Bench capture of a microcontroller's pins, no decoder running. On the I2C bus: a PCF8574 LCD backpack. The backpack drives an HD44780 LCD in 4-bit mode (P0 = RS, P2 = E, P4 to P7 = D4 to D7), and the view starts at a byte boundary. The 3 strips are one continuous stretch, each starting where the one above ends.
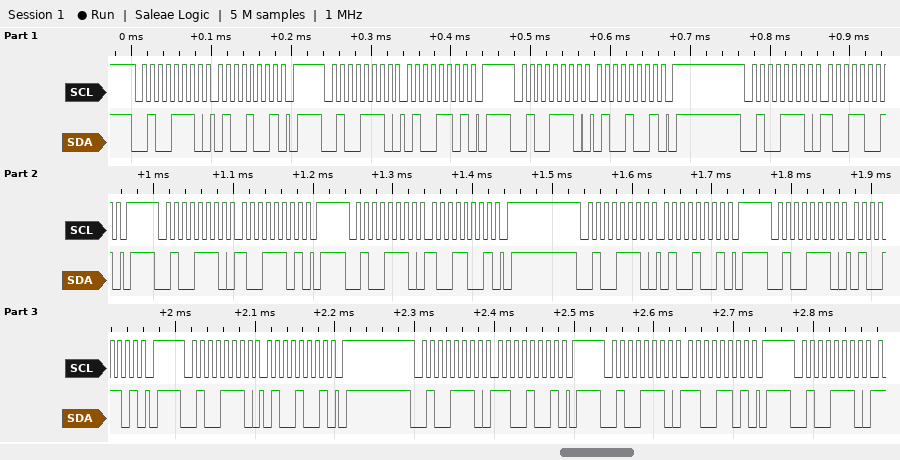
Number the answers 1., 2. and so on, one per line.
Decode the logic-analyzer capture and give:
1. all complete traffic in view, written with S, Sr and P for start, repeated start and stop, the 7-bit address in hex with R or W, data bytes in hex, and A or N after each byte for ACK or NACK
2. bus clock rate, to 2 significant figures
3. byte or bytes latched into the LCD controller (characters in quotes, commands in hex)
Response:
1. S 27W A 49 A P S 27W A 4D A P S 27W A 49 A P S 27W A 99 A P S 27W A 9D A P S 27W A 99 A P S 27W A 49 A P S 27W A 4D A P S 27W A 49 A P S 27W A C9 A P S 27W A CD A P S 27W A
2. 100 kHz
3. 'I'
